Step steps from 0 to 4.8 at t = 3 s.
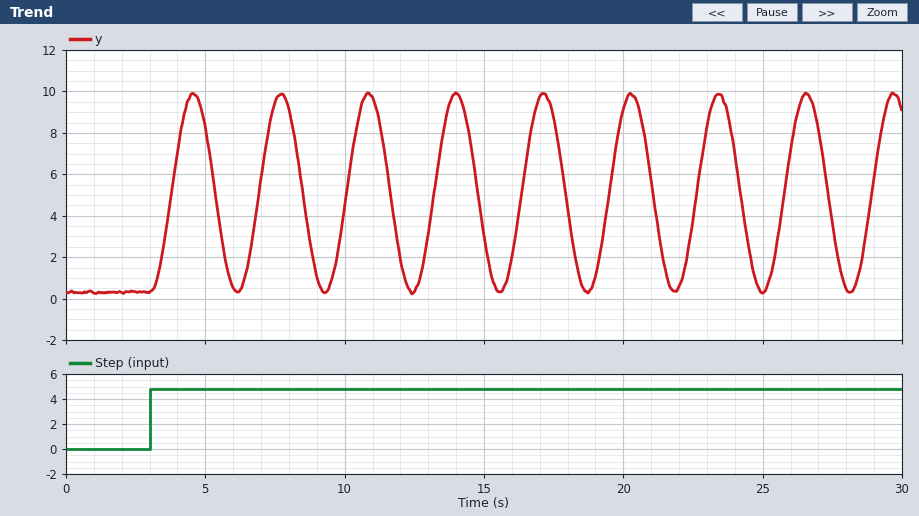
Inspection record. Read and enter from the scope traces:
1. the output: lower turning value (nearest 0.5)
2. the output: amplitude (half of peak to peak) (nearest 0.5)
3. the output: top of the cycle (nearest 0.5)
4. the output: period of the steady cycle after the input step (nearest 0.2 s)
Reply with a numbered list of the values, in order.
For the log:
1. 0.5
2. 5.0
3. 10.0
4. 3.2 s
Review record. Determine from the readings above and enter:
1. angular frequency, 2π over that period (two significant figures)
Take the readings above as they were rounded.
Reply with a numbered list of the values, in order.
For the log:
1. 2.0 rad/s
